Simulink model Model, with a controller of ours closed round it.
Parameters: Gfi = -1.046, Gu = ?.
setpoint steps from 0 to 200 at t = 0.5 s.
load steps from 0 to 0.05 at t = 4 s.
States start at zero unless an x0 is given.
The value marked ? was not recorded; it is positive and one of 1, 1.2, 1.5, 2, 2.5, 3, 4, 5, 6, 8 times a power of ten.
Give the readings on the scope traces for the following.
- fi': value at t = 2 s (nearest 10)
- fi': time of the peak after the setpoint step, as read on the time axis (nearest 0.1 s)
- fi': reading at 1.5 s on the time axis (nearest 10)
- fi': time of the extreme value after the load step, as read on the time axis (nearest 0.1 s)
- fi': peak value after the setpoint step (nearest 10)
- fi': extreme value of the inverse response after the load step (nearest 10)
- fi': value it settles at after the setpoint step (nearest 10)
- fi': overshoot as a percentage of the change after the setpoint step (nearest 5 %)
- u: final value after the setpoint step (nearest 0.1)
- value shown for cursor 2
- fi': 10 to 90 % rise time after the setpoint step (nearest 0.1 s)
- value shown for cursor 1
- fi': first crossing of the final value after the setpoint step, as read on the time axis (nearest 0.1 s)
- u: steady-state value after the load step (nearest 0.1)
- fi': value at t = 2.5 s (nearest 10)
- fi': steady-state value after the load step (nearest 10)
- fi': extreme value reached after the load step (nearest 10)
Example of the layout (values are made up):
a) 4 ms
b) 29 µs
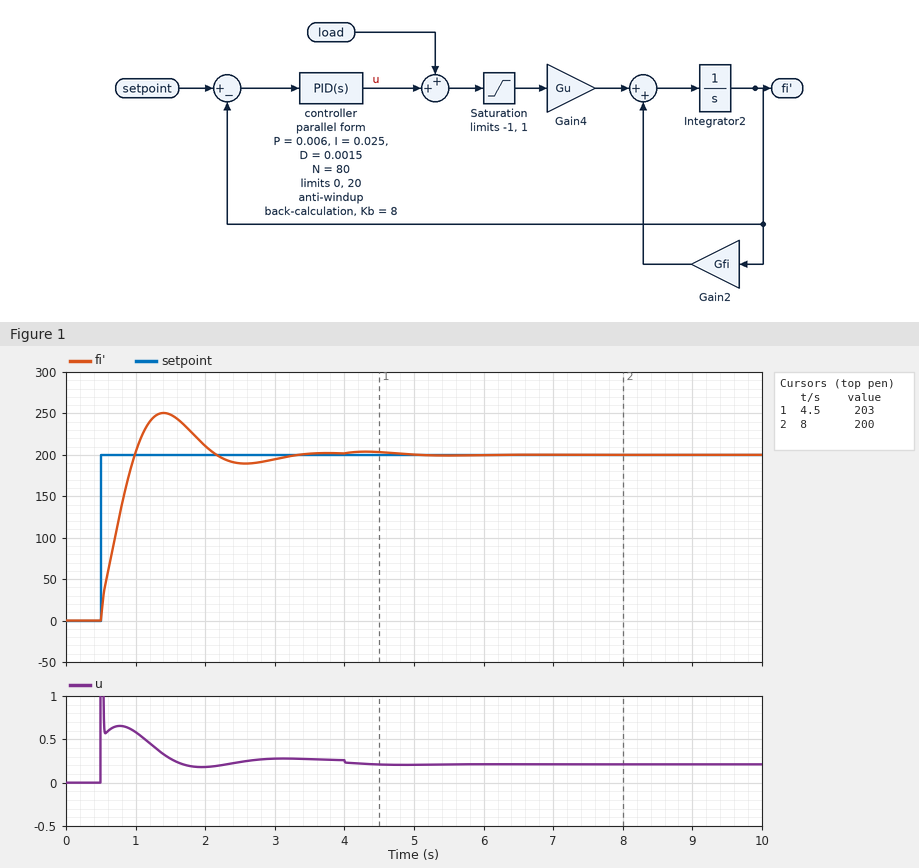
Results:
a) 210
b) 1.4 s
c) 250
d) 5.5 s
e) 250
f) 200
g) 200
h) 25 %
i) 0.3
j) 200
k) 0.4 s
l) 203
m) 1.0 s
n) 0.2
o) 190
p) 200
q) 200
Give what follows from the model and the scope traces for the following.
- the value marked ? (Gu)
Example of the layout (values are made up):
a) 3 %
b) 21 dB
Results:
a) 800
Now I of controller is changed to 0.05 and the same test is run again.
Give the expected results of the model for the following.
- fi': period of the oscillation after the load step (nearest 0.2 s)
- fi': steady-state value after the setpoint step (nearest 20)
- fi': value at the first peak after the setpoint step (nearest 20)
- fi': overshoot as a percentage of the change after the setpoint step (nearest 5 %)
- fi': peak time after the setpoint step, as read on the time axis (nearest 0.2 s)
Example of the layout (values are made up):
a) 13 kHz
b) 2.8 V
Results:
a) 1.6 s
b) 200
c) 280
d) 35 %
e) 1.2 s
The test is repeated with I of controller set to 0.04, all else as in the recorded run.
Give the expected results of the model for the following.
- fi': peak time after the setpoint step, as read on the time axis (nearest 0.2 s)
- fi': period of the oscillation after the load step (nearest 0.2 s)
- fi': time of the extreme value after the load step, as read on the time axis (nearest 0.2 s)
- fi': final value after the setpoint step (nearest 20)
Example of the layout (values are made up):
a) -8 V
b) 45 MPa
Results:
a) 1.2 s
b) 1.8 s
c) 4.4 s
d) 200
